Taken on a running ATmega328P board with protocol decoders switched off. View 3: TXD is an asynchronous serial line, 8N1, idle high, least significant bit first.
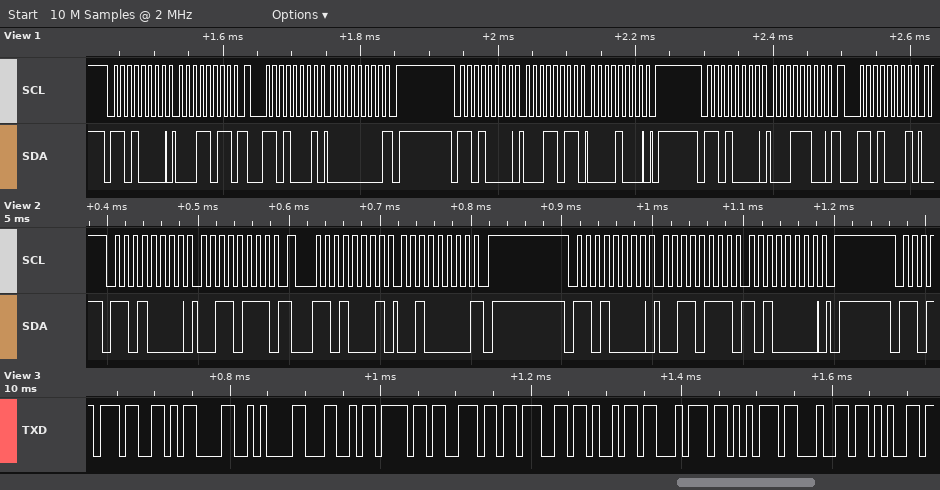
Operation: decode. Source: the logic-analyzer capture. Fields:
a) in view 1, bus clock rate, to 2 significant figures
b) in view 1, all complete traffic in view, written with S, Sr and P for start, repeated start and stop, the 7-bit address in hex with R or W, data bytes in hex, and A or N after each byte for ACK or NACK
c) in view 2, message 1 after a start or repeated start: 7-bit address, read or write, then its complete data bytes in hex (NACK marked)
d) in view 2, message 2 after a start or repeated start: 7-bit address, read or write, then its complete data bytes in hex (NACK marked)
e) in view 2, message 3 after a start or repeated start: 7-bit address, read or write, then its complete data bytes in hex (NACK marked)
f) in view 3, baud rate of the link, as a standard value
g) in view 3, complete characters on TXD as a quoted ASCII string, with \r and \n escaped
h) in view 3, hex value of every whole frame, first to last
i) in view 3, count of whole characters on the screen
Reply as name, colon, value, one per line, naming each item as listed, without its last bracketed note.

in view 1, bus clock rate, to 2 significant figures: 100 kHz
in view 1, all complete traffic in view, written with S, Sr and P for start, repeated start and stop, the 7-bit address in hex with R or W, data bytes in hex, and A or N after each byte for ACK or NACK: S 68W A 1B A Sr 68R A 00 N P S 68W A 1B A 08 A P S 68W A 1C A Sr 68R A
in view 2, message 1 after a start or repeated start: 7-bit address, read or write, then its complete data bytes in hex: 0x68 write: 37
in view 2, message 2 after a start or repeated start: 7-bit address, read or write, then its complete data bytes in hex: 0x68 read: 20 NACK
in view 2, message 3 after a start or repeated start: 7-bit address, read or write, then its complete data bytes in hex: 0x68 write: 37 A0
in view 3, baud rate of the link, as a standard value: 115200 baud
in view 3, complete characters on TXD as a quoted ASCII string, with \r and \n escaped: "7\r\nLongitude"
in view 3, hex value of every whole frame, first to last: 37 0D 0A 4C 6F 6E 67 69 74 75 64 65
in view 3, count of whole characters on the screen: 12
